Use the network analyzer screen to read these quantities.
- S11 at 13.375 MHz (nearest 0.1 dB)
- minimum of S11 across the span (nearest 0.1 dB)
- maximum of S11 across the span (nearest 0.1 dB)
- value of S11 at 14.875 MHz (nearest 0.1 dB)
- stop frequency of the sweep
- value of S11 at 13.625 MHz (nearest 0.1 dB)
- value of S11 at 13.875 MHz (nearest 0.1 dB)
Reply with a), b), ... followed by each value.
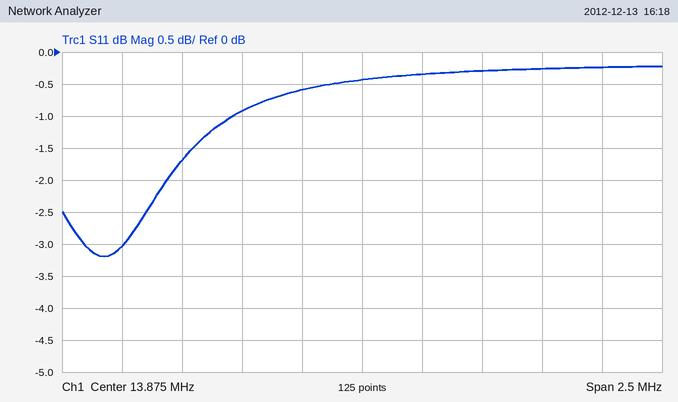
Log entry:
a) -0.9 dB
b) -3.2 dB
c) -0.2 dB
d) -0.2 dB
e) 15.125 MHz
f) -0.6 dB
g) -0.4 dB
